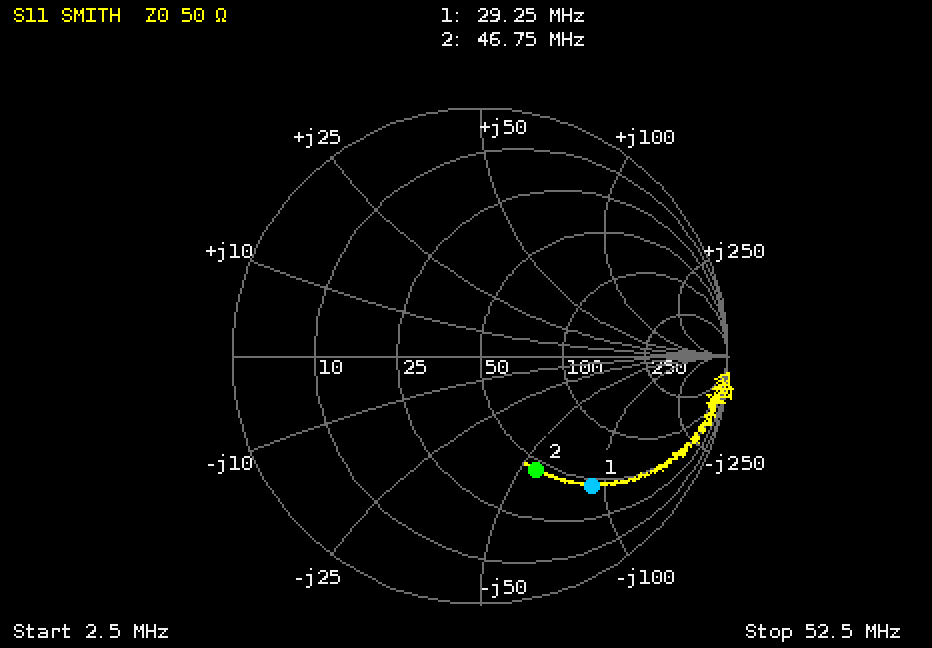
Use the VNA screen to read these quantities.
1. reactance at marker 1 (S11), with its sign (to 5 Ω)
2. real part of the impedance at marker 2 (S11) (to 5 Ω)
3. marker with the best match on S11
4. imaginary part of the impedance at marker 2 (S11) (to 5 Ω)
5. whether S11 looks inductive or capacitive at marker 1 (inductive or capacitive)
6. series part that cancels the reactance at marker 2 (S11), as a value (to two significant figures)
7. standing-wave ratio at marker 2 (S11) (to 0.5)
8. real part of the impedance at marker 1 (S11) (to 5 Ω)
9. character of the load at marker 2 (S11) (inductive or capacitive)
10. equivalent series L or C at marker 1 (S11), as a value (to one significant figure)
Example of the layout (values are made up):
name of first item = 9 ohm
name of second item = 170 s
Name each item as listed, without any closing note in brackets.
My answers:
reactance at marker 1 (S11), with its sign = -90 Ω
real part of the impedance at marker 2 (S11) = 45 Ω
marker with the best match on S11 = marker 2
imaginary part of the impedance at marker 2 (S11) = -55 Ω
whether S11 looks inductive or capacitive at marker 1 = capacitive
series part that cancels the reactance at marker 2 (S11), as a value = 190 nH
standing-wave ratio at marker 2 (S11) = 3.0
real part of the impedance at marker 1 (S11) = 45 Ω
character of the load at marker 2 (S11) = capacitive
equivalent series L or C at marker 1 (S11), as a value = 60 pF
